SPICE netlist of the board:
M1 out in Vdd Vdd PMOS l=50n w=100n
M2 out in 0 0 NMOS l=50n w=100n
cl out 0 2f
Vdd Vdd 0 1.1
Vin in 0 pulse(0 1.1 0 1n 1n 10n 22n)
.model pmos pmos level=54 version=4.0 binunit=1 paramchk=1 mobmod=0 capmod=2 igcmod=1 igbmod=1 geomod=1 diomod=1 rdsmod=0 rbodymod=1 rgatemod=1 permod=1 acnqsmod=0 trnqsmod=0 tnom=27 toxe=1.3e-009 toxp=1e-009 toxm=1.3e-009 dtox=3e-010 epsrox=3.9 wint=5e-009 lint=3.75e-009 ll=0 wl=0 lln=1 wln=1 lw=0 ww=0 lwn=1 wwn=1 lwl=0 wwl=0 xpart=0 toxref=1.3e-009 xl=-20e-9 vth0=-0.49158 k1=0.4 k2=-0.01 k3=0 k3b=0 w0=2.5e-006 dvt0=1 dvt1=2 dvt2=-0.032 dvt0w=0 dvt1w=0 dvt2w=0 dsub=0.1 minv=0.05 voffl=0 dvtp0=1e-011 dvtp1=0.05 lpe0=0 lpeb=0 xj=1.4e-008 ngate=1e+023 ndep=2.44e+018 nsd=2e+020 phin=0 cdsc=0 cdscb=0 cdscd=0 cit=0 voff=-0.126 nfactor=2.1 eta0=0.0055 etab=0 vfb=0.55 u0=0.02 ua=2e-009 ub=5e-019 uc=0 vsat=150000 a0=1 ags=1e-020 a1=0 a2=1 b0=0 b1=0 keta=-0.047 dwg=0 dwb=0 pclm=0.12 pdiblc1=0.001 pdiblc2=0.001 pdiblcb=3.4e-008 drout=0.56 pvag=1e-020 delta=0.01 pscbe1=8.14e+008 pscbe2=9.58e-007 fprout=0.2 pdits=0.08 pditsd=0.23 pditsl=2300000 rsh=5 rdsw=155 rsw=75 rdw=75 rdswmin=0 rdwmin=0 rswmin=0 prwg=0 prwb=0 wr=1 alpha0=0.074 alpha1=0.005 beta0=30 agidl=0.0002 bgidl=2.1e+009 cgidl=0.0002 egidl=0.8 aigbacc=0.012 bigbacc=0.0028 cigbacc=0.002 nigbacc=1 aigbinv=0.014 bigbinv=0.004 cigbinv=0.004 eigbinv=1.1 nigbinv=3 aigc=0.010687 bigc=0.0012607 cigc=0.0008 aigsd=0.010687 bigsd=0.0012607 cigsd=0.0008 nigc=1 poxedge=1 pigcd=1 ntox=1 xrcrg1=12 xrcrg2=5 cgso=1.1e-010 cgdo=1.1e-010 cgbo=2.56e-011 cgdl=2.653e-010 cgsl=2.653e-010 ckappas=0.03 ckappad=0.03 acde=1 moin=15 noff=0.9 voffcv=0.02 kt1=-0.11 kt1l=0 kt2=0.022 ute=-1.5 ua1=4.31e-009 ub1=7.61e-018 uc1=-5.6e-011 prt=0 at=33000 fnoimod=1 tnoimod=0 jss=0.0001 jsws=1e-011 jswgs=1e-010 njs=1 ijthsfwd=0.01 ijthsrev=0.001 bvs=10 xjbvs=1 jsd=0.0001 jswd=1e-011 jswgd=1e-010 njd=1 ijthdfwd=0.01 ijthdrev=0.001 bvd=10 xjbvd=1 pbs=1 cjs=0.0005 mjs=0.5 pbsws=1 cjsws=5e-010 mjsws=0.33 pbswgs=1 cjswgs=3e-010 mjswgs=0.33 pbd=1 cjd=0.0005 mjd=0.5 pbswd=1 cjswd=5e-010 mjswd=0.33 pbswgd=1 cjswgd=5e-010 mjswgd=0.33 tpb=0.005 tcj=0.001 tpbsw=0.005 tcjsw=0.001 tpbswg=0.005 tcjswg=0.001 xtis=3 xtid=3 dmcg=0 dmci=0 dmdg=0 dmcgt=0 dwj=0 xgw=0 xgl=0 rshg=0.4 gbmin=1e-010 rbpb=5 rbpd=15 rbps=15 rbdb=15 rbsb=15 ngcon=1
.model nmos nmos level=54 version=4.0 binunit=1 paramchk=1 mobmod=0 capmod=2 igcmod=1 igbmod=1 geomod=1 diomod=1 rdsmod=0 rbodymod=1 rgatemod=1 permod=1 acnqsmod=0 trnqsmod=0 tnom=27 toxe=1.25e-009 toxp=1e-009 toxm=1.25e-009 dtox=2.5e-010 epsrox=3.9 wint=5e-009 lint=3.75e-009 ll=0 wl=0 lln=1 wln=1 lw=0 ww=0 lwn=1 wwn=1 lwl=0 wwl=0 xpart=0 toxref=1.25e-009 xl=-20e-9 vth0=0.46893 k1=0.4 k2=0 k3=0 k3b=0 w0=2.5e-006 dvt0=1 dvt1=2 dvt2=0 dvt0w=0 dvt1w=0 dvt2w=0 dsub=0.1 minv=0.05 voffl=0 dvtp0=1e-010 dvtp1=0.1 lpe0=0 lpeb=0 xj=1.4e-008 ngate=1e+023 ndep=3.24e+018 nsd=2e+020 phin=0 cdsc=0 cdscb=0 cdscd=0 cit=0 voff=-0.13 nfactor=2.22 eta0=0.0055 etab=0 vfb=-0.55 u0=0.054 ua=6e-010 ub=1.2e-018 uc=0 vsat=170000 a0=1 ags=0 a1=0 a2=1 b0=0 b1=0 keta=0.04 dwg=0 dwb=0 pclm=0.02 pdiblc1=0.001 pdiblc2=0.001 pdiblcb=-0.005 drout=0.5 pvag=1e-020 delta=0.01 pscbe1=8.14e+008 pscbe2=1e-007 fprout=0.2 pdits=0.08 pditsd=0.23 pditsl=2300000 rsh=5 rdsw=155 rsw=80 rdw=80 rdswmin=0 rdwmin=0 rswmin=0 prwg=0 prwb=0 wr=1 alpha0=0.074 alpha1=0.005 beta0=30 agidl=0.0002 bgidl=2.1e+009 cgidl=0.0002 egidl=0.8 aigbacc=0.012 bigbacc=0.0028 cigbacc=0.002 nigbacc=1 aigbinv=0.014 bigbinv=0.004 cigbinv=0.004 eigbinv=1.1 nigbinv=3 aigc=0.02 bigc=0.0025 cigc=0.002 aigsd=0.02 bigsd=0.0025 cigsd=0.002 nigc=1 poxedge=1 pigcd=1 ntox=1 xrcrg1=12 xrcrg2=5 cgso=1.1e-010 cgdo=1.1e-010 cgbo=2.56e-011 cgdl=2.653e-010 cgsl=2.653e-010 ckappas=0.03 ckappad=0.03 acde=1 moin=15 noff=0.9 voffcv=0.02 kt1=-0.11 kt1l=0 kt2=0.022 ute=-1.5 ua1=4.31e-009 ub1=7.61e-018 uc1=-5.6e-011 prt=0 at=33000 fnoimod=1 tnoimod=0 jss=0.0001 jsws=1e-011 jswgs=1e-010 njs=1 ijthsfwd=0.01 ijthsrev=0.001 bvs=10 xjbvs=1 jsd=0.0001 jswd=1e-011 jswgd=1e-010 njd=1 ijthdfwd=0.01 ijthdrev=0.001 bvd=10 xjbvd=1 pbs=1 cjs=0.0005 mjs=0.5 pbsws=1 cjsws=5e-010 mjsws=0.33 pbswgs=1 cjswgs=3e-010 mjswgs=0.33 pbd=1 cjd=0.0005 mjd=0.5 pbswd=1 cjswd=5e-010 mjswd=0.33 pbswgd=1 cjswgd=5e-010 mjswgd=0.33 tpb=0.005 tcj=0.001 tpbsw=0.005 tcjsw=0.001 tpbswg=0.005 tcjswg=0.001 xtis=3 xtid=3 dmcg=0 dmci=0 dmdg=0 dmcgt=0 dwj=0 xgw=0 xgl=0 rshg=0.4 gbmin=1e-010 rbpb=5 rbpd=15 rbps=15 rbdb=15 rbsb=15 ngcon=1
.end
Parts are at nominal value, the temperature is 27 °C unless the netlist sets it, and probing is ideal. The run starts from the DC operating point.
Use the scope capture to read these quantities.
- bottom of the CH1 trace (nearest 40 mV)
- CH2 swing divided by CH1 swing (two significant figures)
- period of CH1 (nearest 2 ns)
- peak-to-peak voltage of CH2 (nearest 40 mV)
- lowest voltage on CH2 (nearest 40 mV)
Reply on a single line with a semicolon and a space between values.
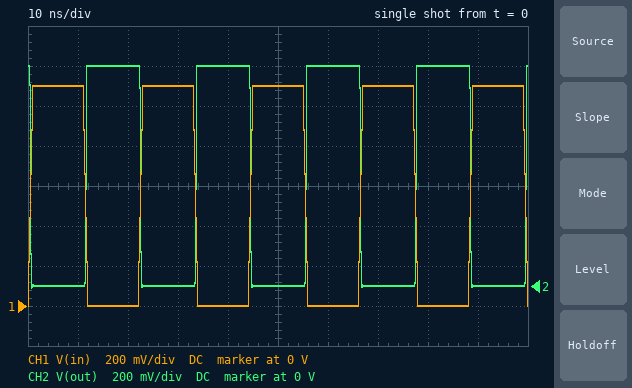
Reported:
0 V; 1.0; 22 ns; 1.12 V; 0 V
